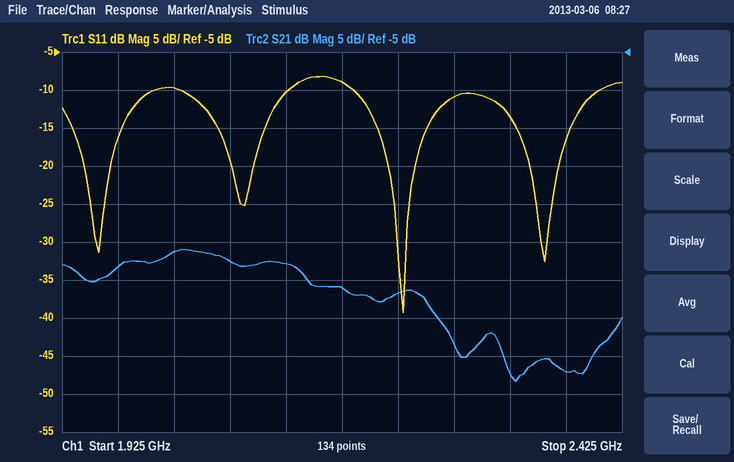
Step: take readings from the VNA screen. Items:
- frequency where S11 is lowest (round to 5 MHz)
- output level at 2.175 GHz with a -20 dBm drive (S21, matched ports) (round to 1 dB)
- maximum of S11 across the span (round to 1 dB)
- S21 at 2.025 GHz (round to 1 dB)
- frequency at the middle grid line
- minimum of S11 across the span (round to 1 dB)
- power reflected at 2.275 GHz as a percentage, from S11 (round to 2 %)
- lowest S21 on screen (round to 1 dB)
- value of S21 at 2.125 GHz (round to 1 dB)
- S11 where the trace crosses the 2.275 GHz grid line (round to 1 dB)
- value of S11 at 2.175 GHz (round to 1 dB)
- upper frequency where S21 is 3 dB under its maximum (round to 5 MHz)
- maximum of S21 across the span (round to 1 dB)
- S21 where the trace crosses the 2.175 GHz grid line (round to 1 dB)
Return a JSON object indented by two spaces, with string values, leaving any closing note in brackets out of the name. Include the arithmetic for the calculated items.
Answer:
{
  "frequency where S11 is lowest": "2.230 GHz",
  "output level at 2.175 GHz with a -20 dBm drive (S21, matched ports)": "-20 dBm + (-36 dB) = -56 dBm",
  "maximum of S11 across the span": "-8 dB",
  "S21 at 2.025 GHz": "-31 dB",
  "frequency at the middle grid line": "2.175 GHz",
  "minimum of S11 across the span": "-39 dB",
  "power reflected at 2.275 GHz as a percentage, from S11": "10^(-11/10) ≈ 8 %",
  "lowest S21 on screen": "-48 dB",
  "value of S21 at 2.125 GHz": "-33 dB",
  "S11 where the trace crosses the 2.275 GHz grid line": "-11 dB",
  "value of S11 at 2.175 GHz": "-9 dB",
  "upper frequency where S21 is 3 dB under its maximum": "2.140 GHz",
  "maximum of S21 across the span": "-31 dB",
  "S21 where the trace crosses the 2.175 GHz grid line": "-36 dB"
}
